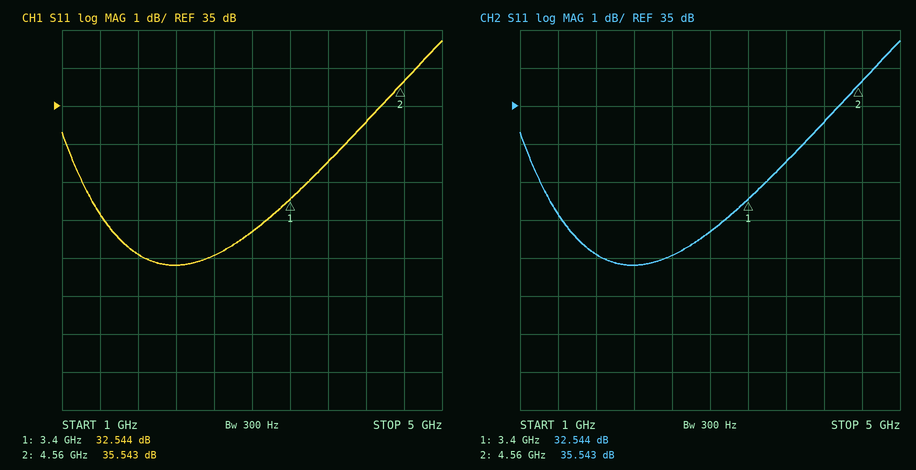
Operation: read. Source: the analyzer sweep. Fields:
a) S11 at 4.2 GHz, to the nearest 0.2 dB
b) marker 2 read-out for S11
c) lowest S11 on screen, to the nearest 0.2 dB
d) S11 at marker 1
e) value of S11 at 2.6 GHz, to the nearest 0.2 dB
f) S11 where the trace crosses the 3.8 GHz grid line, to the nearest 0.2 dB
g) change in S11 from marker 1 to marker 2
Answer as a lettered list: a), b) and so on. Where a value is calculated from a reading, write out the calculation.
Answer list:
a) 34.6 dB
b) 35.543 dB
c) 30.8 dB
d) 32.544 dB
e) 31.0 dB
f) 33.6 dB
g) 35.543 − (32.544) = 2.999 dB
